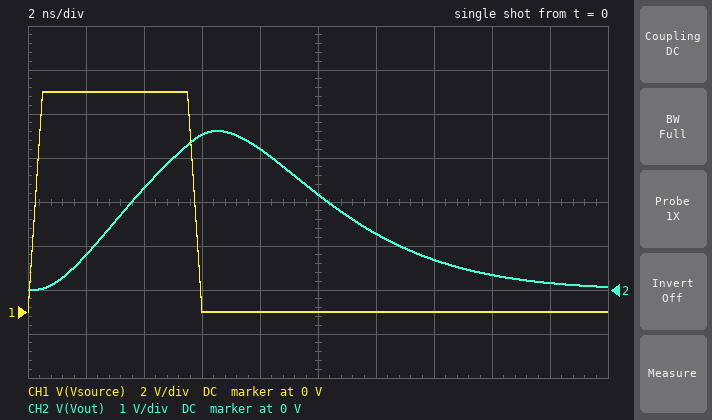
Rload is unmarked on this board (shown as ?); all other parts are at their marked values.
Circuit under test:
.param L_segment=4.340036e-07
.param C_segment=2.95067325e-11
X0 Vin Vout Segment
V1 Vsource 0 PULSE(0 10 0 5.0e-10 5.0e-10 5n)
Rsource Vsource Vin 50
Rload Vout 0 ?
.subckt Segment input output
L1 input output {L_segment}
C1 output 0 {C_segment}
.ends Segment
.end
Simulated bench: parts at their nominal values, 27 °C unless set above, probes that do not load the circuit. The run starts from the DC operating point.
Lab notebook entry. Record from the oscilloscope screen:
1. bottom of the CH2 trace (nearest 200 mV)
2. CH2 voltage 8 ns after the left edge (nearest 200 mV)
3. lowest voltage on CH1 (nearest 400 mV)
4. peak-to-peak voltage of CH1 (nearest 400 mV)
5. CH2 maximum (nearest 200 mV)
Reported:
0 V
3.2 V
0 V
10.0 V
3.6 V
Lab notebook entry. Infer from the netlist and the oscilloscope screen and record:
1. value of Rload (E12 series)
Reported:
56 Ω
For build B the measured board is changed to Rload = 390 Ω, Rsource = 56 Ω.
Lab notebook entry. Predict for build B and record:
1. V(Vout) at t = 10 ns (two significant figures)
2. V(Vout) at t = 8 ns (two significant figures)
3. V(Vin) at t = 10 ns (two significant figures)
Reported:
6.4 V
8.0 V
1.1 V
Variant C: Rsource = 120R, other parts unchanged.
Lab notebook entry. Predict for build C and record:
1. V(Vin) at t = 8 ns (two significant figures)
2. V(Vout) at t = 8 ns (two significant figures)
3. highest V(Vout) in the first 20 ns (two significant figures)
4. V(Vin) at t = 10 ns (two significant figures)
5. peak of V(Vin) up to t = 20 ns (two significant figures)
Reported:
-2.4 V
2.0 V
2.6 V
-780 mV
9.3 V
